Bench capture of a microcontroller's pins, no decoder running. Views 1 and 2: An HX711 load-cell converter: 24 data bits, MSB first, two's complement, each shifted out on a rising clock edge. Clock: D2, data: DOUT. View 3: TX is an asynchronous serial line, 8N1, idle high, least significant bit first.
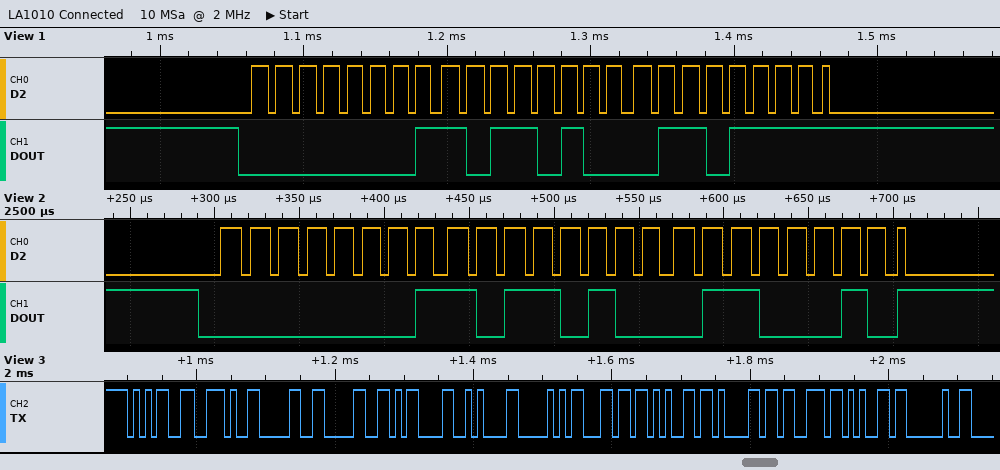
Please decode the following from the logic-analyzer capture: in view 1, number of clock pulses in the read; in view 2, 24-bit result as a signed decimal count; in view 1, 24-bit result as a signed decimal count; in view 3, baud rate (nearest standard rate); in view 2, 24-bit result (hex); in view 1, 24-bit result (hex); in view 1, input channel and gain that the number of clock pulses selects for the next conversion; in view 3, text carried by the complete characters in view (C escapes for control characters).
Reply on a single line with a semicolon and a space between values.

25; 111714; 111727; 115200 baud; 0x01B462; 0x01B46F; channel A, gain 128; "5.00\r\nPlease "
